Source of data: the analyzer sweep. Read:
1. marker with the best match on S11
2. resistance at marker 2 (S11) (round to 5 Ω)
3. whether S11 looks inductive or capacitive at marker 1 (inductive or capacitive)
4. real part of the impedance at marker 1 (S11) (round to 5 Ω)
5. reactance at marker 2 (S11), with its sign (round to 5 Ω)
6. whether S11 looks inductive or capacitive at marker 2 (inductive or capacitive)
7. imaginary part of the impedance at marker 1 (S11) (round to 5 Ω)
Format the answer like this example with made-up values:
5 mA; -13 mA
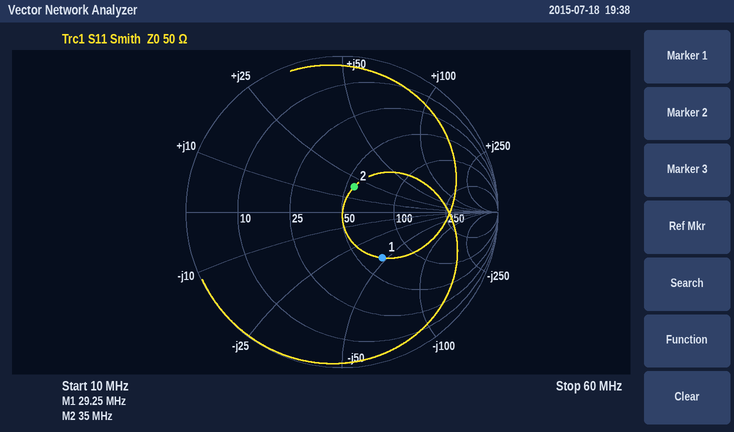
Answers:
marker 2; 55 Ω; capacitive; 65 Ω; +20 Ω; inductive; -45 Ω
